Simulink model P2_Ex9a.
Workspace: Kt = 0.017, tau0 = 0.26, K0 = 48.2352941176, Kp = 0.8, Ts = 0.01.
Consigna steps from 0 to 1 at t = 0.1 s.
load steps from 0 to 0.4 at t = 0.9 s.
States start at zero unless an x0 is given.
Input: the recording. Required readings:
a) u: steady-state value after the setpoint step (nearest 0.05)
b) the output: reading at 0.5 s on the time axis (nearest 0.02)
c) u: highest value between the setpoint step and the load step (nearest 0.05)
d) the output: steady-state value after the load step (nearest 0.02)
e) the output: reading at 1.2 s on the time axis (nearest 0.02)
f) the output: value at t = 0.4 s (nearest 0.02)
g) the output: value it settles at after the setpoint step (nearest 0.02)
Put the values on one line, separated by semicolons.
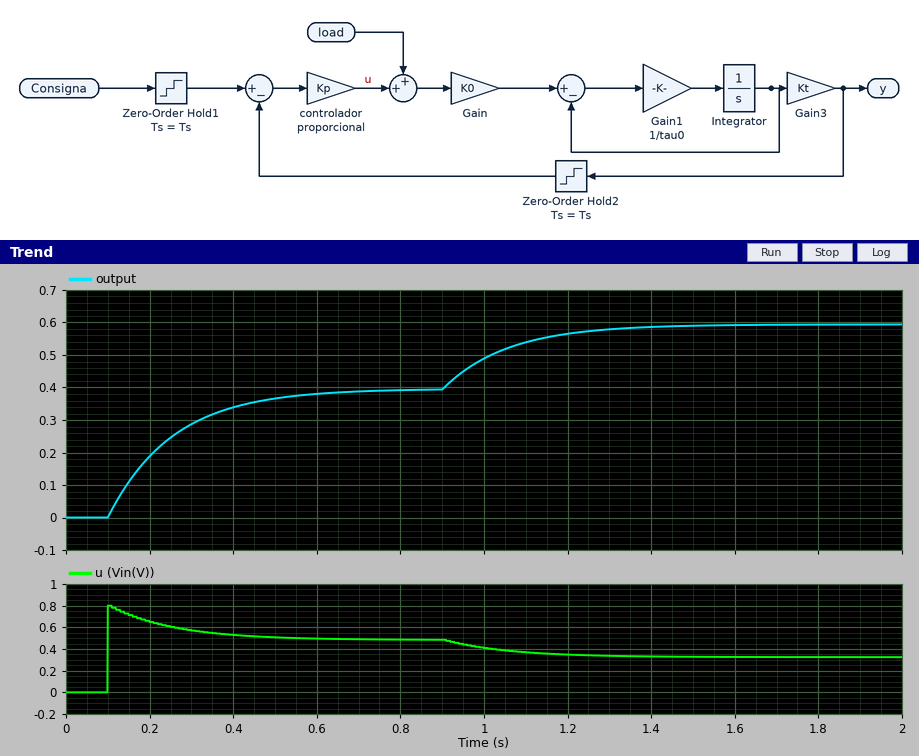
0.50; 0.36; 0.80; 0.60; 0.56; 0.34; 0.40
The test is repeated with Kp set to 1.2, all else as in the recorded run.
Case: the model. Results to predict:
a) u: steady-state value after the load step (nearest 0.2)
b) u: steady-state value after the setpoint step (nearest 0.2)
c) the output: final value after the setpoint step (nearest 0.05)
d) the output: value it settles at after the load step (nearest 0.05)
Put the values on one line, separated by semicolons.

0.4; 0.6; 0.50; 0.65
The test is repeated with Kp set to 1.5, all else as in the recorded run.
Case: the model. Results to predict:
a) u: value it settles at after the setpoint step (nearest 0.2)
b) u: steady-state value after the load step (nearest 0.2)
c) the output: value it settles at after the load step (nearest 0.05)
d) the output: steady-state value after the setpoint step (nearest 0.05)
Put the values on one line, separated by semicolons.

0.6; 0.4; 0.70; 0.55
